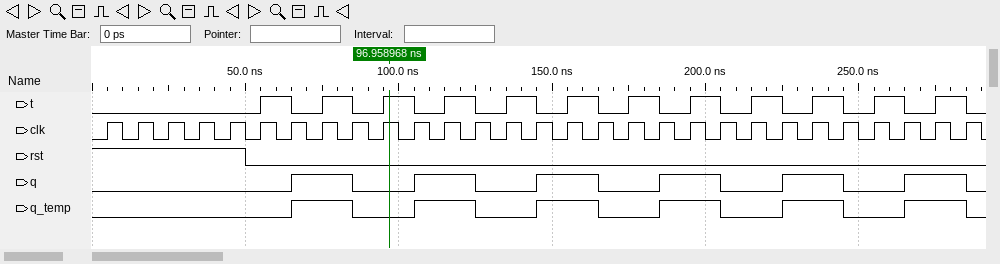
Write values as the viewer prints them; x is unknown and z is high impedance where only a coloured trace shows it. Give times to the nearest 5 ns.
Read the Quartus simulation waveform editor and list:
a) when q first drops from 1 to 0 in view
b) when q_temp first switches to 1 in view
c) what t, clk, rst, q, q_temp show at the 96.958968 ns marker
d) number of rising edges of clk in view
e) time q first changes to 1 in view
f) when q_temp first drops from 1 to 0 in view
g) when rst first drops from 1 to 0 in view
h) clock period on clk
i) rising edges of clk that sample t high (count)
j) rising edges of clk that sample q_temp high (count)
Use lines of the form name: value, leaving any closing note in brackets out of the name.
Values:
when q first drops from 1 to 0 in view: 85 ns
when q_temp first switches to 1 in view: 65 ns
what t, clk, rst, q, q_temp show at the 96.958968 ns marker: t=1, clk=1, rst=0, q=0, q_temp=0
number of rising edges of clk in view: 29
time q first changes to 1 in view: 65 ns
when q_temp first drops from 1 to 0 in view: 85 ns
when rst first drops from 1 to 0 in view: 50 ns
clock period on clk: 10 ns
rising edges of clk that sample t high: 12
rising edges of clk that sample q_temp high: 12
